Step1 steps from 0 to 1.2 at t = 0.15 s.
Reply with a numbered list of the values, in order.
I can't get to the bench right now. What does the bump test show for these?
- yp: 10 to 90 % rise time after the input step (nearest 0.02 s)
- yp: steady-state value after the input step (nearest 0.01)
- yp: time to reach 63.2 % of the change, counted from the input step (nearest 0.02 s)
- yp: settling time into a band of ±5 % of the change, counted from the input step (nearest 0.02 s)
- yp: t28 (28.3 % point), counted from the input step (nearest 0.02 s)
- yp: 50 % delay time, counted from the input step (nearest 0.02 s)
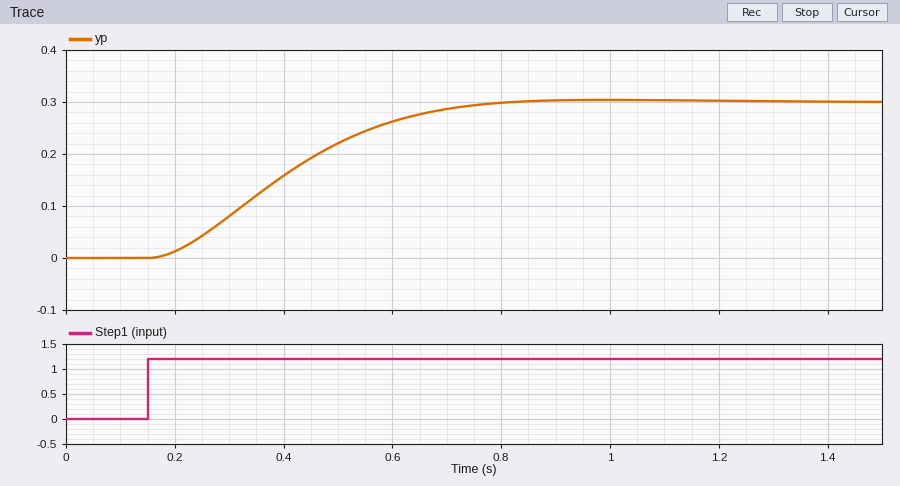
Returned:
1. 0.40 s
2. 0.30
3. 0.30 s
4. 0.54 s
5. 0.16 s
6. 0.24 s
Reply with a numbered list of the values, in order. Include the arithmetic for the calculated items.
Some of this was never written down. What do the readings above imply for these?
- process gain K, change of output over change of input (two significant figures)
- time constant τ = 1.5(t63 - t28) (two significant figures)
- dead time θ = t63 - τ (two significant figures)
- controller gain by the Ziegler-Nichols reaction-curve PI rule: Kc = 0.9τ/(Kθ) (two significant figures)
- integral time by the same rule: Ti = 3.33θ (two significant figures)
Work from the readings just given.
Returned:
1. (0.3 - 0) / 1.2 = 0.25
2. 1.5 × (0.3 - 0.16) = 0.21 s
3. 0.3 - 0.21 = 0.090 s
4. 0.9 × 0.21 / (0.25 × 0.09) = 8.4
5. 3.33 × 0.09 = 0.30 s
